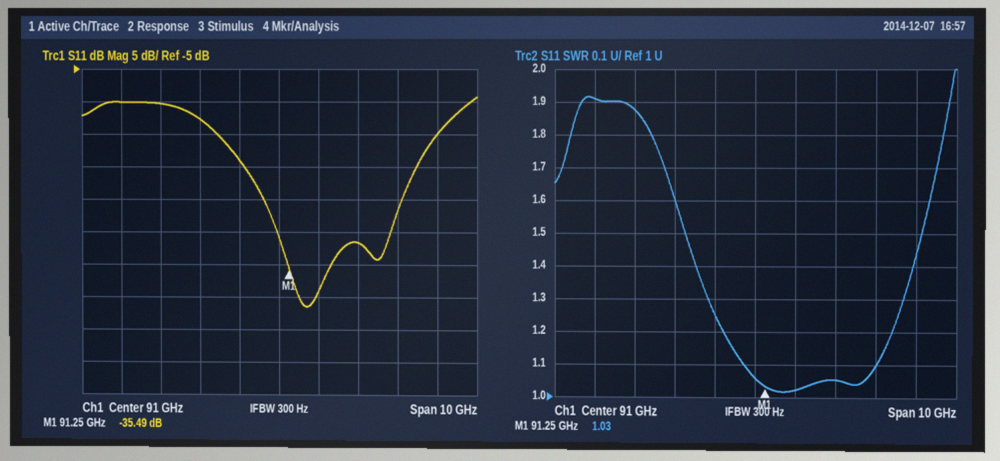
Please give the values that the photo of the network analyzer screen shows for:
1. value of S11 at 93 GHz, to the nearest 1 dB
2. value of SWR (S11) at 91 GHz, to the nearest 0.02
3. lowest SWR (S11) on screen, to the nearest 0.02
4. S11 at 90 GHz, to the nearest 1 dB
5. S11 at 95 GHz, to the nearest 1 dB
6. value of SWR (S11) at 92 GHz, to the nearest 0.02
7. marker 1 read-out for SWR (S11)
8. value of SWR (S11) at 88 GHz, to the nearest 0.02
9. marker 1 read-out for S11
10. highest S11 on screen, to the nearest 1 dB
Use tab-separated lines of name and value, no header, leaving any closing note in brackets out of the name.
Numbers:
value of S11 at 93 GHz, to the nearest 1 dB	-32 dB
value of SWR (S11) at 91 GHz, to the nearest 0.02	1.06
lowest SWR (S11) on screen, to the nearest 0.02	1.02
S11 at 90 GHz, to the nearest 1 dB	-19 dB
S11 at 95 GHz, to the nearest 1 dB	-15 dB
value of SWR (S11) at 92 GHz, to the nearest 0.02	1.02
marker 1 read-out for SWR	1.03
value of SWR (S11) at 88 GHz, to the nearest 0.02	1.88
marker 1 read-out for S11	-35.49 dB
highest S11 on screen, to the nearest 1 dB	-9 dB
